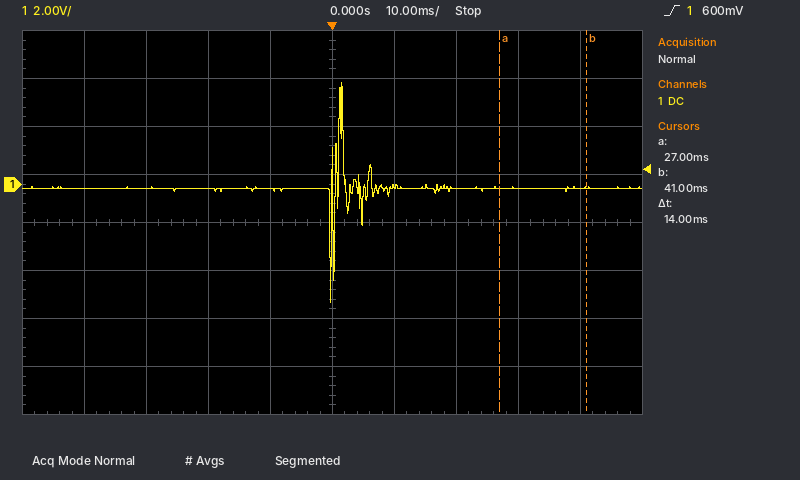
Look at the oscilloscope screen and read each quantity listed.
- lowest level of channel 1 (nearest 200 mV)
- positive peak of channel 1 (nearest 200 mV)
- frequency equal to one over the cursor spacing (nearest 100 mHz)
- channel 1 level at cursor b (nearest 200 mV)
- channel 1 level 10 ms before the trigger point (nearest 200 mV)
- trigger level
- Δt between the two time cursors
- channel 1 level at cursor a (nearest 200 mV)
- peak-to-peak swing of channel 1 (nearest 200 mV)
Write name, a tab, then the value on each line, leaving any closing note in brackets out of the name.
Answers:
lowest level of channel 1	-5.0 V
positive peak of channel 1	4.2 V
frequency equal to one over the cursor spacing	71.4 Hz
channel 1 level at cursor b	-200 mV
channel 1 level 10 ms before the trigger point	-200 mV
trigger level	600 mV
Δt between the two time cursors	14 ms
channel 1 level at cursor a	-200 mV
peak-to-peak swing of channel 1	9.2 V
